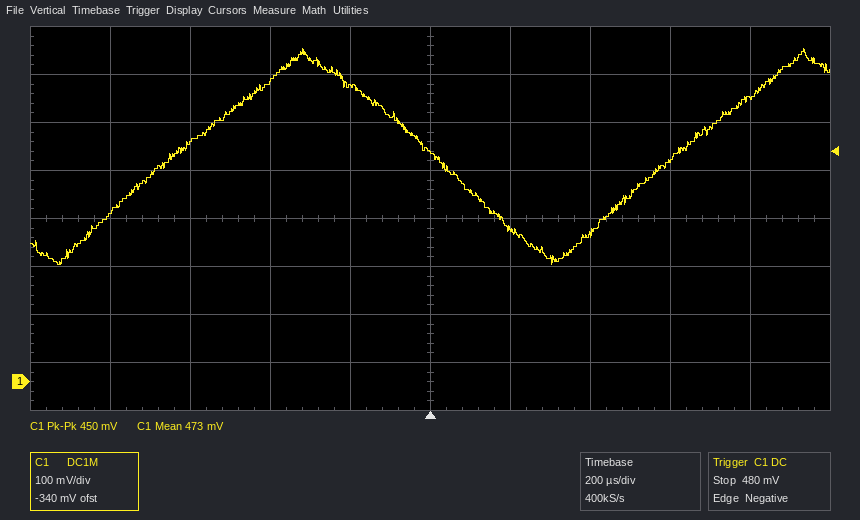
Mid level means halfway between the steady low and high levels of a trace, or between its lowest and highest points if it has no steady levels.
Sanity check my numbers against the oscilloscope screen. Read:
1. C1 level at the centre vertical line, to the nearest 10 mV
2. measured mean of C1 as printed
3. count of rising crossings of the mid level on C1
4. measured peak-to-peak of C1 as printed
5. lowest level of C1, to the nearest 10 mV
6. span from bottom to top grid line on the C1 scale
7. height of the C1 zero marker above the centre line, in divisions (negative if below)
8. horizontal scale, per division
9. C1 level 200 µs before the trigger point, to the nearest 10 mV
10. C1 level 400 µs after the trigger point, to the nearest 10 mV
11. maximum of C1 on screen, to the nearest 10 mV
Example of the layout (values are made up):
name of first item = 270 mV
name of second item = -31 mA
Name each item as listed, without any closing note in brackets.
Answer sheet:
C1 level at the centre vertical line, to the nearest 10 mV = 480 mV
measured mean of C1 as printed = 473 mV
count of rising crossings of the mid level on C1 = 2
measured peak-to-peak of C1 as printed = 450 mV
lowest level of C1, to the nearest 10 mV = 240 mV
span from bottom to top grid line on the C1 scale = 800 mV
height of the C1 zero marker above the centre line, in divisions = -3.4 div
horizontal scale, per division = 200 µs
C1 level 200 µs before the trigger point, to the nearest 10 mV = 620 mV
C1 level 400 µs after the trigger point, to the nearest 10 mV = 310 mV
maximum of C1 on screen, to the nearest 10 mV = 690 mV
